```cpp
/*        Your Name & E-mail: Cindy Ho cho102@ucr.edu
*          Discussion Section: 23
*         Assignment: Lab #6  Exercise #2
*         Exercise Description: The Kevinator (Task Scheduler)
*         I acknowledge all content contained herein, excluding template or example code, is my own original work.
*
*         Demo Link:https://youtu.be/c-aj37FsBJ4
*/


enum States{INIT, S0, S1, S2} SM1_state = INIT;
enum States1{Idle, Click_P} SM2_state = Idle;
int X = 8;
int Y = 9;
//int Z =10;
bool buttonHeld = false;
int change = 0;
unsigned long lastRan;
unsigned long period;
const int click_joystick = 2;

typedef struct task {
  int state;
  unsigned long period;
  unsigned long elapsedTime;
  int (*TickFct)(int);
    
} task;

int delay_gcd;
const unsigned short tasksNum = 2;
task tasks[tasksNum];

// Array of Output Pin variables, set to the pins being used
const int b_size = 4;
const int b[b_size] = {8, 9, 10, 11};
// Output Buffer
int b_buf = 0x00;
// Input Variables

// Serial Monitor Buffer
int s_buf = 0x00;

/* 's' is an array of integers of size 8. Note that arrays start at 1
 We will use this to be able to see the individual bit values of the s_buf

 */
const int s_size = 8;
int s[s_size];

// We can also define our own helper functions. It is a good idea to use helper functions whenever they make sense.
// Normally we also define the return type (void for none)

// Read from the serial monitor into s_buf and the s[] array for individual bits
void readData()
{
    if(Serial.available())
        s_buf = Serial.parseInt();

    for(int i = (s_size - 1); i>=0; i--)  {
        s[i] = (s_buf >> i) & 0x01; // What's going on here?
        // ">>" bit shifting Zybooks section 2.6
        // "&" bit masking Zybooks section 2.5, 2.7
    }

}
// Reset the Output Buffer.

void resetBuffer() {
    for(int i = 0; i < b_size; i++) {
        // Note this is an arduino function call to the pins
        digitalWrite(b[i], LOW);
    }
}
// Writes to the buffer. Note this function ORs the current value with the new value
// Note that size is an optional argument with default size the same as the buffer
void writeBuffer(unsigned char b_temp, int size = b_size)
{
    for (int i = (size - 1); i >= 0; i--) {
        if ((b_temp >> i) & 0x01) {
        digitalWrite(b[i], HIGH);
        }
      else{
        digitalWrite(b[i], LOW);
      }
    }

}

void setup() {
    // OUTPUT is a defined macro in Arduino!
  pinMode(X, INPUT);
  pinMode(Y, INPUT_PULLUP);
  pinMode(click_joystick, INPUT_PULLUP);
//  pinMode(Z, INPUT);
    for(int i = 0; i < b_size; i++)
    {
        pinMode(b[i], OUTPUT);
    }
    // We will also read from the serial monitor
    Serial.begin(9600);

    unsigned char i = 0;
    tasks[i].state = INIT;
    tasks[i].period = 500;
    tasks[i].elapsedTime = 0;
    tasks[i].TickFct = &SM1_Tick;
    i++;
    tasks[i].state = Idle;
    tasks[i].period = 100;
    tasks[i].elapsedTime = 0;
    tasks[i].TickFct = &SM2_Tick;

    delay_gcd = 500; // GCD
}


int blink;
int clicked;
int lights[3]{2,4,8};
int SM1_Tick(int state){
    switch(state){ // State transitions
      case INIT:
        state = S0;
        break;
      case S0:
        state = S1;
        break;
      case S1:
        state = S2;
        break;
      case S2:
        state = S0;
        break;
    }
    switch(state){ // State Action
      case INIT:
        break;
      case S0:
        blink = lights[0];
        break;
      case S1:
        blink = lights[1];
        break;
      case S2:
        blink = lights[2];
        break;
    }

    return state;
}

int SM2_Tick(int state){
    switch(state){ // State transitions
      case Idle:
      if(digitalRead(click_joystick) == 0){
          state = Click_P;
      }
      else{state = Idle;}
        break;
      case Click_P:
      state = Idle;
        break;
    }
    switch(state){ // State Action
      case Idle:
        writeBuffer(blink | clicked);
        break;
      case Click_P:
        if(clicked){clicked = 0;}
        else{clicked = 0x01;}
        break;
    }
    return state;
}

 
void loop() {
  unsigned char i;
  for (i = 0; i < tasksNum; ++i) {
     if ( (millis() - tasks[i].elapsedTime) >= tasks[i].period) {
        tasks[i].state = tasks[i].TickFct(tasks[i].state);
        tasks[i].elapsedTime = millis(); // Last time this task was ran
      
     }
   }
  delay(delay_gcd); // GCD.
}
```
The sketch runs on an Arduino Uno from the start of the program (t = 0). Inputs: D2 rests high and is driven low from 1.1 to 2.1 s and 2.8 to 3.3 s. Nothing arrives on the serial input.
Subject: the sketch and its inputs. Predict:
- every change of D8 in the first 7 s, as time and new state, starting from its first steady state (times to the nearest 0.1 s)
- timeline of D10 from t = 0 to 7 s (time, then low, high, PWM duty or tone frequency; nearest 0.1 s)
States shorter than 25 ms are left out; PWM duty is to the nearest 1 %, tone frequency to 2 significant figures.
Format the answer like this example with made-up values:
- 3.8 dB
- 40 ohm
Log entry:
- 0 s low; 2 s high; 3.5 s low
- 0 s low; 2 s high; 2.5 s low; 3.5 s high; 4.5 s low; 6 s high; 6.5 s low
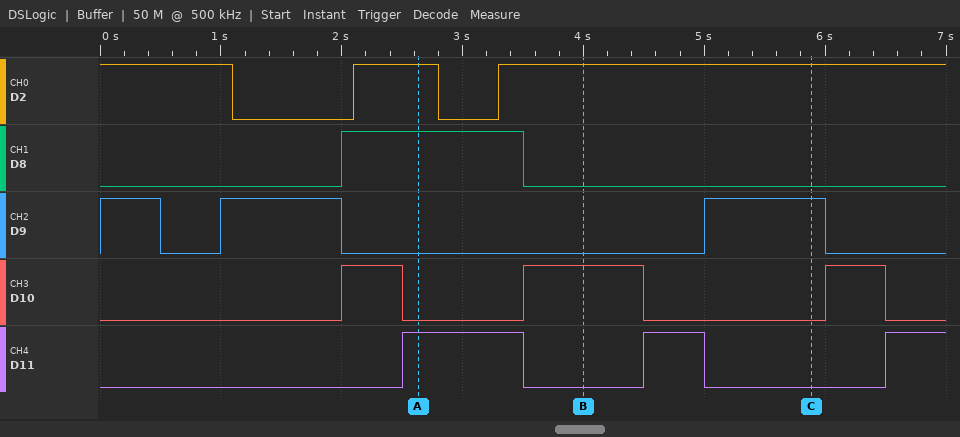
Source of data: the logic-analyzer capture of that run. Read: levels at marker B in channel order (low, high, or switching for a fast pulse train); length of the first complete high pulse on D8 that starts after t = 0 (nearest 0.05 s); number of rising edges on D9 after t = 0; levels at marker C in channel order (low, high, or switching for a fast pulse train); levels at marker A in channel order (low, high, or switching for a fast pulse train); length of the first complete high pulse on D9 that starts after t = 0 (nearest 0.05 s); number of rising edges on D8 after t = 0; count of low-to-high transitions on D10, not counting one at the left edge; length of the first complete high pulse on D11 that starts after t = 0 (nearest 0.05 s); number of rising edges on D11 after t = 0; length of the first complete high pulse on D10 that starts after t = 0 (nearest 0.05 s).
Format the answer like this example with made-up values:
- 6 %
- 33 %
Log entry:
- D2 high, D8 low, D9 low, D10 high, D11 low
- 1.50 s
- 2
- D2 high, D8 low, D9 high, D10 low, D11 low
- D2 high, D8 high, D9 low, D10 low, D11 high
- 1.00 s
- 1
- 3
- 1.00 s
- 3
- 0.50 s
